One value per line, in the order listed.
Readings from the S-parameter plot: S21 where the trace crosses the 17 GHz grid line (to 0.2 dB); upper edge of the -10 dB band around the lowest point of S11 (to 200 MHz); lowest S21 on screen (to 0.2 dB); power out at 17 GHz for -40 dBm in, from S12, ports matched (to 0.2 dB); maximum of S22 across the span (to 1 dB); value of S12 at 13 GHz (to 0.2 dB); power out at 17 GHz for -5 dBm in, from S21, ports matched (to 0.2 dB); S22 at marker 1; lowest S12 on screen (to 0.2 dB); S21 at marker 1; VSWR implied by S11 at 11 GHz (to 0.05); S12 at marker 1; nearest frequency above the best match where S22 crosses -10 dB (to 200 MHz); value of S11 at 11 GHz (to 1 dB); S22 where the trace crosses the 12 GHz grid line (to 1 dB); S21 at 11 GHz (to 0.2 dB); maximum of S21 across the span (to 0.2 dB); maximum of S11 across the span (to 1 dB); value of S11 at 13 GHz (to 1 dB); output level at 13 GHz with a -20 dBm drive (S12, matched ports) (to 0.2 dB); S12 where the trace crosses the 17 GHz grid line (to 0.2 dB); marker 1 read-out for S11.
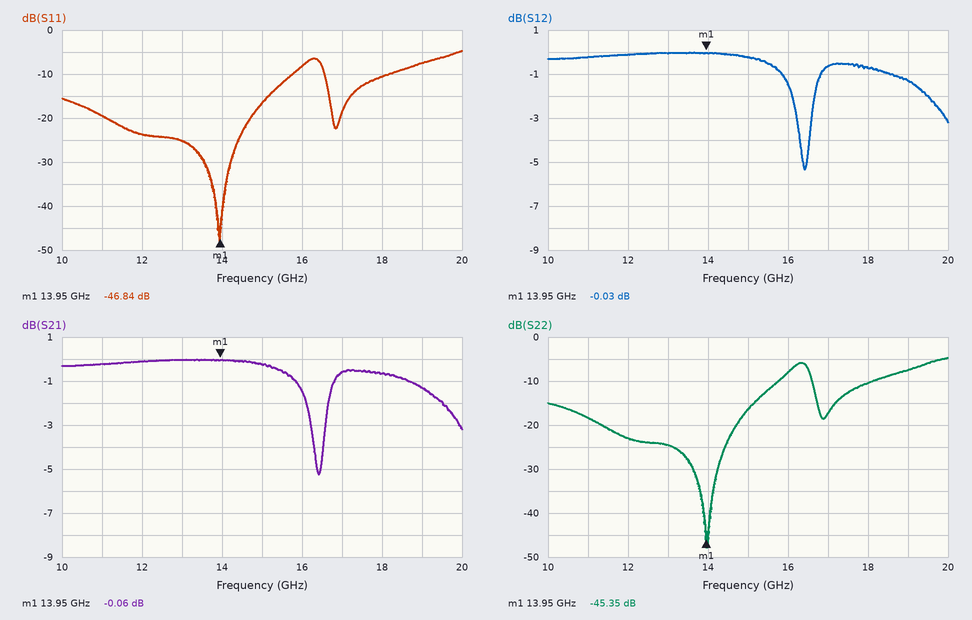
-0.6 dB
15.8 GHz
-5.2 dB
-40.6 dBm
-5 dB
0.0 dB
-5.6 dBm
-45.35 dB
-5.4 dB
-0.06 dB
1.25
-0.03 dB
15.8 GHz
-19 dB
-23 dB
-0.2 dB
0.0 dB
-5 dB
-25 dB
-20.0 dBm
-0.6 dB
-46.84 dB
